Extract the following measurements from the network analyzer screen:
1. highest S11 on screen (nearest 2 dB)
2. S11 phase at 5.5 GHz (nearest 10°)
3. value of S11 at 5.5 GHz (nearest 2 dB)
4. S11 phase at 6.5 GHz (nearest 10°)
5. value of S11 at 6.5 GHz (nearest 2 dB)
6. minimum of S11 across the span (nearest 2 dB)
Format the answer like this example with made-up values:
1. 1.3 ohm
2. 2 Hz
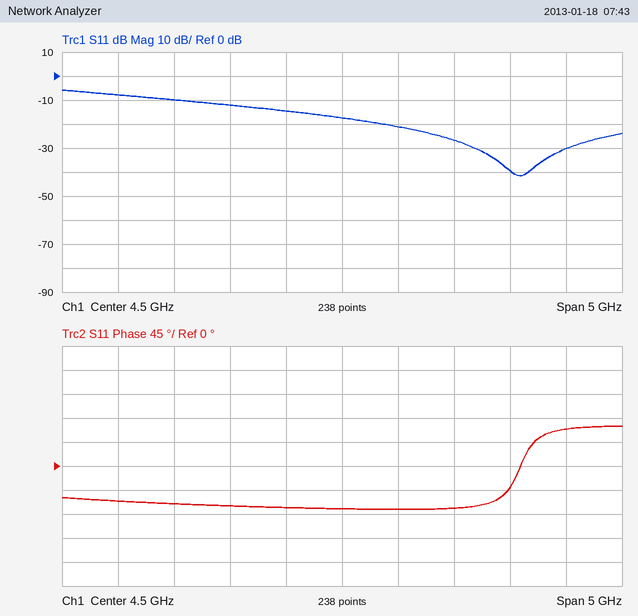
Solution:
1. -6 dB
2. -80°
3. -26 dB
4. 70°
5. -30 dB
6. -42 dB
